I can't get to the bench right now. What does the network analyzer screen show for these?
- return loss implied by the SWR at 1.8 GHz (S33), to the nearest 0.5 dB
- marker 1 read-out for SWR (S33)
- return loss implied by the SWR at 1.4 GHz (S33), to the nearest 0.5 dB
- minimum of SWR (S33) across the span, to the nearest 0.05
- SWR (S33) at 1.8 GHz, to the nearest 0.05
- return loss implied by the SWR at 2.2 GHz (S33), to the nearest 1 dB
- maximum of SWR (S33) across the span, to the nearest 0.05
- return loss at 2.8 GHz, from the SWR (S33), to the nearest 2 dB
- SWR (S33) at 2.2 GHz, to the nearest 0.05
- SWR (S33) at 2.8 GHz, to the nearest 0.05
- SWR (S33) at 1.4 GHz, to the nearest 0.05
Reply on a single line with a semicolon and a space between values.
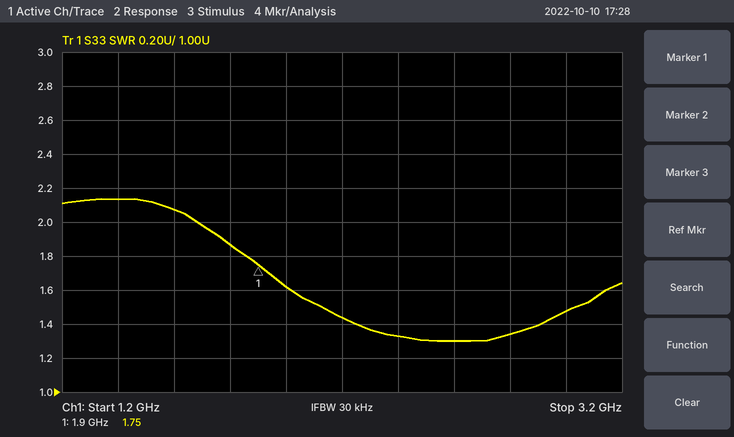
10.5 dB; 1.75; 9.0 dB; 1.30; 1.85; 15 dB; 2.15; 16 dB; 1.45; 1.35; 2.15
